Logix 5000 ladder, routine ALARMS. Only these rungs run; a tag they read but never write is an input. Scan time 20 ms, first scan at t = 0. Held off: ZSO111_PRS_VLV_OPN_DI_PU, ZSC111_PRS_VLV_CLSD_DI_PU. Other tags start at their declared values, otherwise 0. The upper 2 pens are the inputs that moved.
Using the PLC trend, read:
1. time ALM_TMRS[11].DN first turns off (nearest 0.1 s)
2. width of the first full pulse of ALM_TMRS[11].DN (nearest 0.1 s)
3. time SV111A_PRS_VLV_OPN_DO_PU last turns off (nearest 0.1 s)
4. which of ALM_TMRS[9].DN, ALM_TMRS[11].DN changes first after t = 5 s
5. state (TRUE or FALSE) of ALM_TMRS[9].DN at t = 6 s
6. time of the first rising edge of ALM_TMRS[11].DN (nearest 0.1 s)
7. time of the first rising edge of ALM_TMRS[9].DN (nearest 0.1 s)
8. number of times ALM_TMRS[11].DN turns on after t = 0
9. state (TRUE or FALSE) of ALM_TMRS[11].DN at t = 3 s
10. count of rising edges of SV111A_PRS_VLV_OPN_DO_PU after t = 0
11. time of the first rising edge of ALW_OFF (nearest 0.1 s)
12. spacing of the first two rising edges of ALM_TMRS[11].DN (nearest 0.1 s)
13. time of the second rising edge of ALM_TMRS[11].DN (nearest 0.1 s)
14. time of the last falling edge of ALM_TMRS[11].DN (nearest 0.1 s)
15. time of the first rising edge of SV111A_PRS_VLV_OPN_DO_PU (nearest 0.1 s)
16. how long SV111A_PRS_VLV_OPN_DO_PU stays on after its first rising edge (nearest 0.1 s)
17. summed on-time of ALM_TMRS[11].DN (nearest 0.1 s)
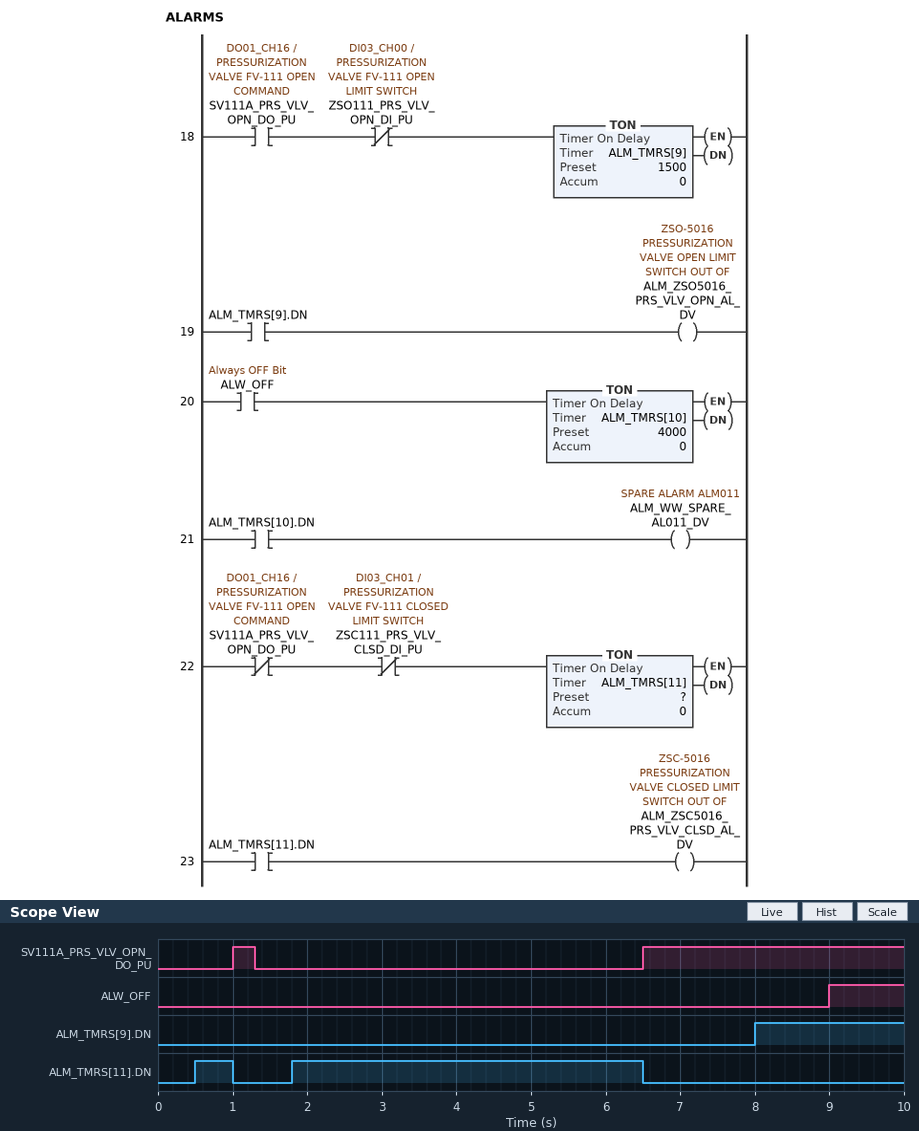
1.0 s
0.5 s
1.3 s
ALM_TMRS[11].DN
FALSE
0.5 s
8.0 s
2
TRUE
2
9.0 s
1.3 s
1.8 s
6.5 s
1.0 s
0.3 s
5.2 s
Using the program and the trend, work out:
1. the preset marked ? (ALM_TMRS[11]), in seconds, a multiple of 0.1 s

0.5 s
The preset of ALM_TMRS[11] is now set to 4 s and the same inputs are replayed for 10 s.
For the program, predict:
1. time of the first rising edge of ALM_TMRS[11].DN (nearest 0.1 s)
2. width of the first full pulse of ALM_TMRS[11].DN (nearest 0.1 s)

5.3 s
1.2 s
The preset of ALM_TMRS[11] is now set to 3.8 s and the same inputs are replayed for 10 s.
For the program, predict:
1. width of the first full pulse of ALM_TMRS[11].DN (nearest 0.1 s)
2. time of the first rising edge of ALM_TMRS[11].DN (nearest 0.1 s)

1.4 s
5.1 s
